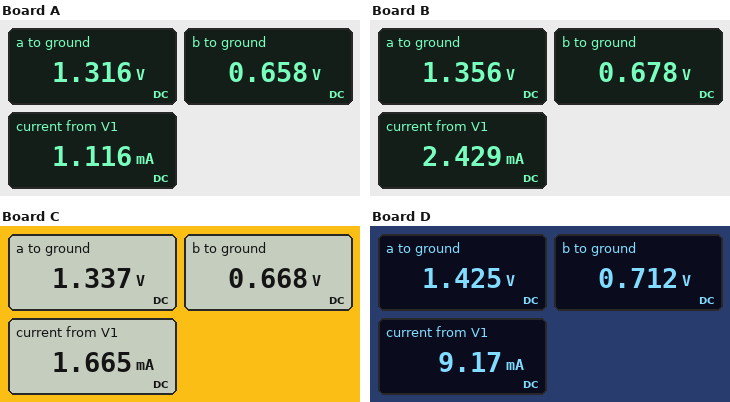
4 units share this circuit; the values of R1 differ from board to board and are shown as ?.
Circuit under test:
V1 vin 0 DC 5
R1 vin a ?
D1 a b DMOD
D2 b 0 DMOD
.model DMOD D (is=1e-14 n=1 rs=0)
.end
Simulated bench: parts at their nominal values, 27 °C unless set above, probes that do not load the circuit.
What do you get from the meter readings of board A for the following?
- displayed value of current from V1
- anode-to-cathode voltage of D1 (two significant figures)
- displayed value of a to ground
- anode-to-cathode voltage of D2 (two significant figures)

1.116 mA
660 mV
1.316 V
660 mV
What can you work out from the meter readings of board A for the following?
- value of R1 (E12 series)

3.3 kΩ
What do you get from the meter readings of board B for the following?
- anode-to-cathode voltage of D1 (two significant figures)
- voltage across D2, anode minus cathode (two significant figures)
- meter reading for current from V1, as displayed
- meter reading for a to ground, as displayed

680 mV
680 mV
2.429 mA
1.356 V
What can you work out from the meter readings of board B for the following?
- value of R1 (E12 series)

1.5 kΩ
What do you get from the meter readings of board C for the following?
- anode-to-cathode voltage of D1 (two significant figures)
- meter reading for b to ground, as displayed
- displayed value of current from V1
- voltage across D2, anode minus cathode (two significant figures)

670 mV
0.668 V
1.665 mA
670 mV
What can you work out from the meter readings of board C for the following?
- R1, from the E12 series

2.2 kΩ
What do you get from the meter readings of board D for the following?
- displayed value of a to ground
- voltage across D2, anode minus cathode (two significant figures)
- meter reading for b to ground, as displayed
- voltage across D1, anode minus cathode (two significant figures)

1.425 V
710 mV
0.712 V
710 mV
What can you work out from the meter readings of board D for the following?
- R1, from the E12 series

390 Ω
